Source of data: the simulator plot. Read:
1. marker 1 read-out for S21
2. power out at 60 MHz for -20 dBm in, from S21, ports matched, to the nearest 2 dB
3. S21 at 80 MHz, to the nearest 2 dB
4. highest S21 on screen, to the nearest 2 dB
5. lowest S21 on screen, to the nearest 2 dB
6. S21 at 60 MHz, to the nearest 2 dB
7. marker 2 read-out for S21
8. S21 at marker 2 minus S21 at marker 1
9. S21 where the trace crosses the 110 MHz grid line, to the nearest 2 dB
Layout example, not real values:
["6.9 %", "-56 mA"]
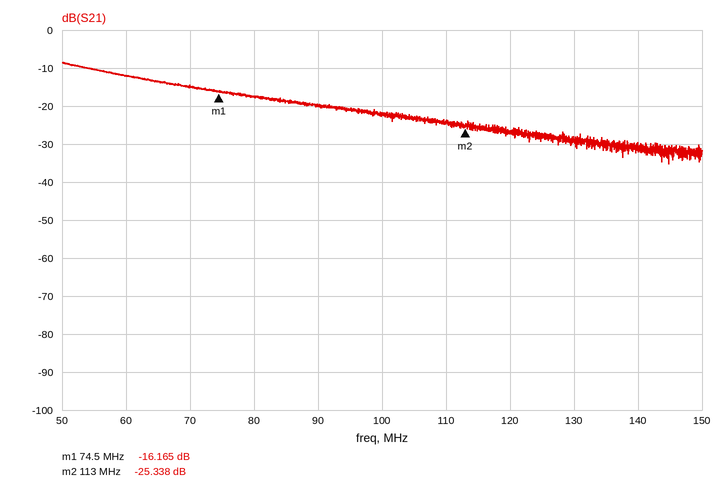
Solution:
["-16.165 dB", "-32 dBm", "-18 dB", "-8 dB", "-36 dB", "-12 dB", "-25.338 dB", "-9.173 dB", "-24 dB"]
